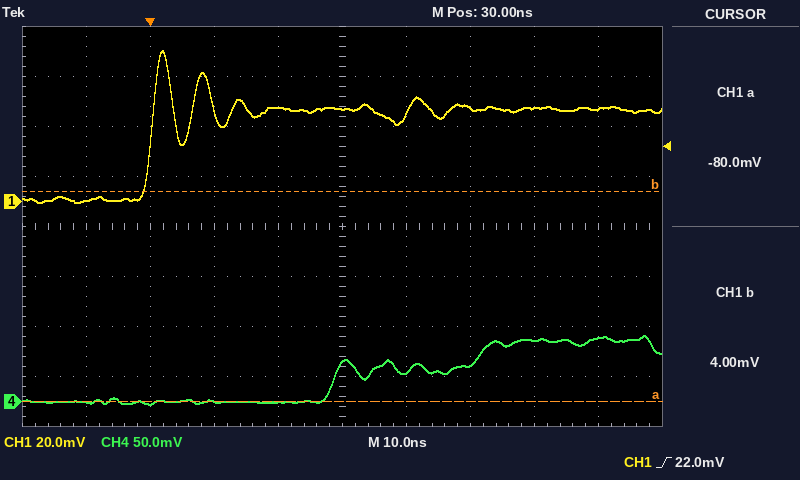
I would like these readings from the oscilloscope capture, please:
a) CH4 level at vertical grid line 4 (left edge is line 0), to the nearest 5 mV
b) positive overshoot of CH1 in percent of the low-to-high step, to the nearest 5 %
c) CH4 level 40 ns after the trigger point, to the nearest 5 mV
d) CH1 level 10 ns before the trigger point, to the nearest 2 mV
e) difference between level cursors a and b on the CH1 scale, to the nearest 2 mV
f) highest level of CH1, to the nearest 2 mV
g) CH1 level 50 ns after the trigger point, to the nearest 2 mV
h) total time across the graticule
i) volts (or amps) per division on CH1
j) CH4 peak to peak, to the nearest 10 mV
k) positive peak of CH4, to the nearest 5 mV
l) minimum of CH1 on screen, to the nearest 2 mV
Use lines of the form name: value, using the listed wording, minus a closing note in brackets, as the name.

CH4 level at vertical grid line 4 (left edge is line 0), to the nearest 5 mV: 0 mV
positive overshoot of CH1 in percent of the low-to-high step, to the nearest 5 %: 65 %
CH4 level 40 ns after the trigger point, to the nearest 5 mV: 30 mV
CH1 level 10 ns before the trigger point, to the nearest 2 mV: 0 mV
difference between level cursors a and b on the CH1 scale, to the nearest 2 mV: 84 mV
highest level of CH1, to the nearest 2 mV: 60 mV
CH1 level 50 ns after the trigger point, to the nearest 2 mV: 38 mV
total time across the graticule: 100 ns
volts (or amps) per division on CH1: 20 mV
CH4 peak to peak, to the nearest 10 mV: 70 mV
positive peak of CH4, to the nearest 5 mV: 65 mV
minimum of CH1 on screen, to the nearest 2 mV: 0 mV
